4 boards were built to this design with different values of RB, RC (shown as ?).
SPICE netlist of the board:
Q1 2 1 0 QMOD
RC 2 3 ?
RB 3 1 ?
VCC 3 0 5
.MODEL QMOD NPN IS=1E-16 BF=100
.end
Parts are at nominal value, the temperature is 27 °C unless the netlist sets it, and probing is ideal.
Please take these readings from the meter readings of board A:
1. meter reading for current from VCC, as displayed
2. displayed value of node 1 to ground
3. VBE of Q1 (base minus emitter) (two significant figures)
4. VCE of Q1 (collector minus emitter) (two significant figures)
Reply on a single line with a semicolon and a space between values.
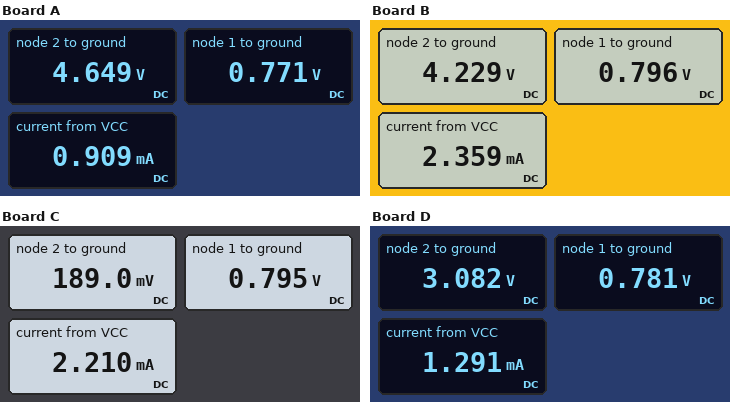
0.909 mA; 0.771 V; 770 mV; 4.6 V
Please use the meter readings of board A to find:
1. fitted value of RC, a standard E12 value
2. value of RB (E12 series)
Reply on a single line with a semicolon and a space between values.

390 Ω; 470 kΩ
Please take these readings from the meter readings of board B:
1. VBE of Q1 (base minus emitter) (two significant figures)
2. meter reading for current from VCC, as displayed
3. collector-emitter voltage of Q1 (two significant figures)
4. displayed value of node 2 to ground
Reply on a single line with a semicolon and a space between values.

800 mV; 2.359 mA; 4.2 V; 4.229 V
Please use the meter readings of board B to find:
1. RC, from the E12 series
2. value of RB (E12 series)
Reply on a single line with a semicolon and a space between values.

330 Ω; 180 kΩ
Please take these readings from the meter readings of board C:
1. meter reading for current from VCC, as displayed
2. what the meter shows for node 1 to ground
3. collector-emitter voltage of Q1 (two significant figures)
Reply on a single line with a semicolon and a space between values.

2.210 mA; 0.795 V; 190 mV
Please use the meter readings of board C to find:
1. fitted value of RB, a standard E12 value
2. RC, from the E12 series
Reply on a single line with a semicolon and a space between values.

180 kΩ; 2.2 kΩ
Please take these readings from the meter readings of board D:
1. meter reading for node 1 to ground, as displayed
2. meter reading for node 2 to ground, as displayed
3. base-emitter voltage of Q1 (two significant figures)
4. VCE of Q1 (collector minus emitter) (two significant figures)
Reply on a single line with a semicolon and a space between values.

0.781 V; 3.082 V; 780 mV; 3.1 V
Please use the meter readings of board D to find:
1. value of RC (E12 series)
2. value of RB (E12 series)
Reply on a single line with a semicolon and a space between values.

1.5 kΩ; 330 kΩ
